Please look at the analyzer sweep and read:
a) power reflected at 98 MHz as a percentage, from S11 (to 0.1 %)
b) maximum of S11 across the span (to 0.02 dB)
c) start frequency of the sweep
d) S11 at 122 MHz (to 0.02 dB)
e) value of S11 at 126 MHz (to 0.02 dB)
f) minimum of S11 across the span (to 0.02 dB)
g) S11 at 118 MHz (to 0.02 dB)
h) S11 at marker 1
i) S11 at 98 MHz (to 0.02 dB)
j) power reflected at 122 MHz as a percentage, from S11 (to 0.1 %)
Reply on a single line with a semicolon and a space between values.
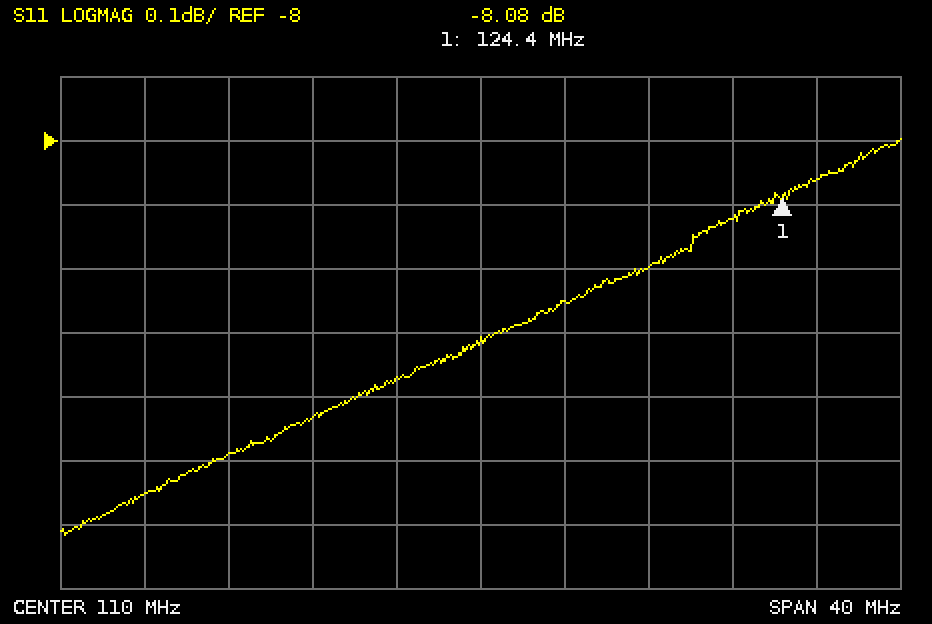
14.2 %; -8.00 dB; 90 MHz; -8.12 dB; -8.06 dB; -8.62 dB; -8.20 dB; -8.08 dB; -8.48 dB; 15.4 %
